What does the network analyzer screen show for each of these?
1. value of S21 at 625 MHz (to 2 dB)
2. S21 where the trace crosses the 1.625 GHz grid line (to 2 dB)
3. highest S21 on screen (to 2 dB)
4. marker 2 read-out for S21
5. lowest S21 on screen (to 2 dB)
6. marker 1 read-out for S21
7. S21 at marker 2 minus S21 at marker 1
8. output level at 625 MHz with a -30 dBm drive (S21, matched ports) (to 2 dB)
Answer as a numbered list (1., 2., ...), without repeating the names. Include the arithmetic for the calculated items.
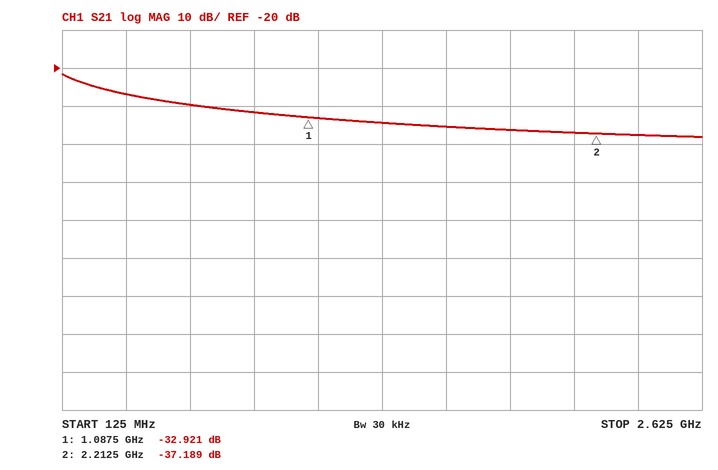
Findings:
1. -30 dB
2. -36 dB
3. -22 dB
4. -37.189 dB
5. -38 dB
6. -32.921 dB
7. -37.189 − (-32.921) = -4.268 dB
8. -30 dBm + (-30 dB) = -60 dBm
